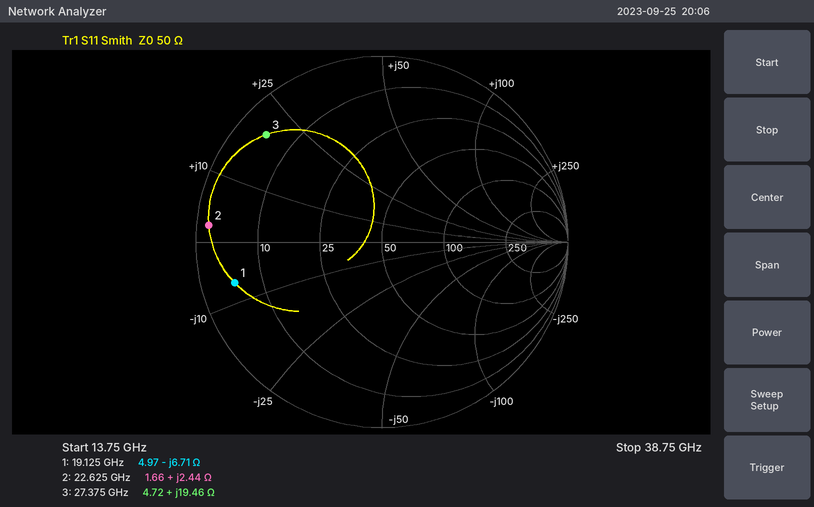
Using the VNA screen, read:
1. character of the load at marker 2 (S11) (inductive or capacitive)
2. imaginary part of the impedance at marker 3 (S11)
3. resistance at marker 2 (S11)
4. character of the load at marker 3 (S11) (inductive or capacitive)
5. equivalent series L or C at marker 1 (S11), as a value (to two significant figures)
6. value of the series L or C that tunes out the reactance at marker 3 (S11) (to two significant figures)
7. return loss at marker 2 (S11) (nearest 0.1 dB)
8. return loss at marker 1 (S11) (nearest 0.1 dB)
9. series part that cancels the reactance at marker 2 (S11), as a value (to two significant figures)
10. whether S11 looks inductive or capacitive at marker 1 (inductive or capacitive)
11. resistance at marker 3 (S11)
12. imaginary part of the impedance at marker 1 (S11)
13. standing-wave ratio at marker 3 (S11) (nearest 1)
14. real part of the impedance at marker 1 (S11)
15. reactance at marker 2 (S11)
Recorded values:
inductive
+19.46 Ω
1.66 Ω
inductive
1.2 pF
300 fF
0.6 dB
1.7 dB
2.9 pF
capacitive
4.72 Ω
-6.71 Ω
12
4.97 Ω
+2.44 Ω
